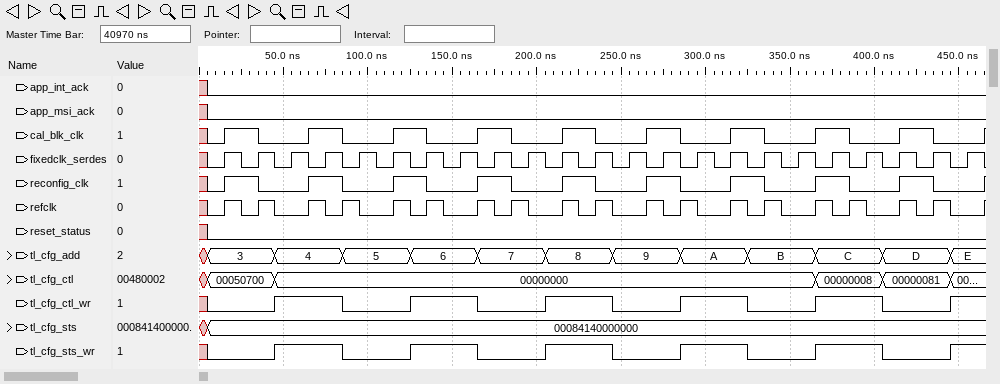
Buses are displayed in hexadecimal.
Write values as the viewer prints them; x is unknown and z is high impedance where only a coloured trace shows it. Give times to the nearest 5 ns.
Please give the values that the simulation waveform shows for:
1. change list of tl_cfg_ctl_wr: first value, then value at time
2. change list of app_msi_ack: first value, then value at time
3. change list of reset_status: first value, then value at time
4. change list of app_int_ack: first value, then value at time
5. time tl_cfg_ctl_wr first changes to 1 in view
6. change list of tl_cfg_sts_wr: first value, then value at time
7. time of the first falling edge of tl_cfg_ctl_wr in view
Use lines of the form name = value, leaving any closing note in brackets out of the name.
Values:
change list of tl_cfg_ctl_wr: first value, then value at time = x, 0 at 5 ns, 1 at 45 ns, 0 at 85 ns, 1 at 125 ns, 0 at 165 ns, 1 at 205 ns, 0 at 245 ns, 1 at 285 ns, 0 at 325 ns, 1 at 365 ns, 0 at 405 ns, 1 at 445 ns
change list of app_msi_ack: first value, then value at time = x, 0 at 5 ns
change list of reset_status: first value, then value at time = x, 0 at 5 ns
change list of app_int_ack: first value, then value at time = x, 0 at 5 ns
time tl_cfg_ctl_wr first changes to 1 in view = 45 ns
change list of tl_cfg_sts_wr: first value, then value at time = x, 0 at 5 ns, 1 at 45 ns, 0 at 85 ns, 1 at 125 ns, 0 at 165 ns, 1 at 205 ns, 0 at 245 ns, 1 at 285 ns, 0 at 325 ns, 1 at 365 ns, 0 at 405 ns, 1 at 445 ns
time of the first falling edge of tl_cfg_ctl_wr in view = 85 ns
